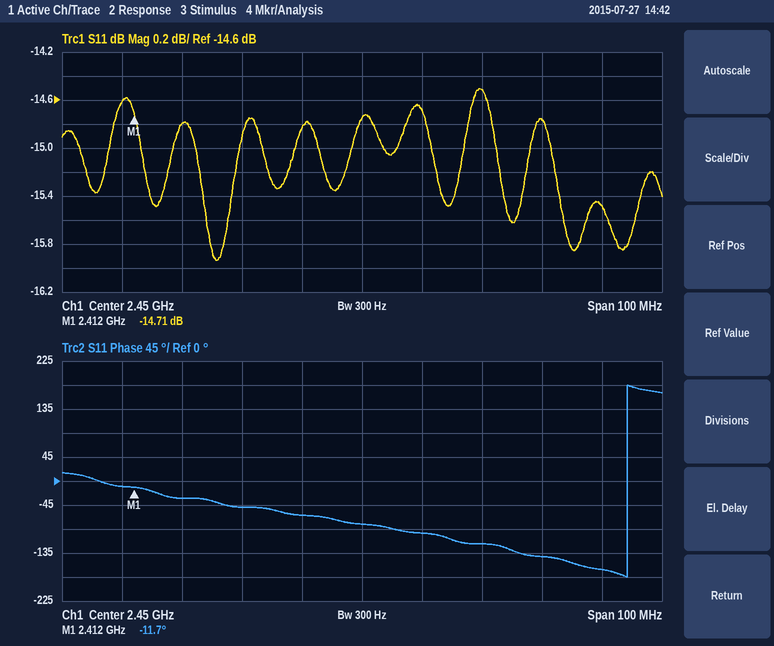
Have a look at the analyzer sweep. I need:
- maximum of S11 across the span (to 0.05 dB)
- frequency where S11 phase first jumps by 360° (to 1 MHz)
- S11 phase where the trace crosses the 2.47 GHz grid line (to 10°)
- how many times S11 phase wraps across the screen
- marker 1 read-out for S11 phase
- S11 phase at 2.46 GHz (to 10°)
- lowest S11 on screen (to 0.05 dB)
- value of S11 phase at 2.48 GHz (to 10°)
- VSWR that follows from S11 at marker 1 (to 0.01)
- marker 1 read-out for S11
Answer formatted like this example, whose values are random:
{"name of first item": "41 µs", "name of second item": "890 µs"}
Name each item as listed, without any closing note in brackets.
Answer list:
{"maximum of S11 across the span": "-14.50 dB", "frequency where S11 phase first jumps by 360°": "2.494 GHz", "S11 phase where the trace crosses the 2.47 GHz grid line": "-120°", "how many times S11 phase wraps across the screen": "1", "marker 1 read-out for S11 phase": "-11.7°", "S11 phase at 2.46 GHz": "-100°", "lowest S11 on screen": "-15.95 dB", "value of S11 phase at 2.48 GHz": "-140°", "VSWR that follows from S11 at marker 1": "1.45", "marker 1 read-out for S11": "-14.71 dB"}
